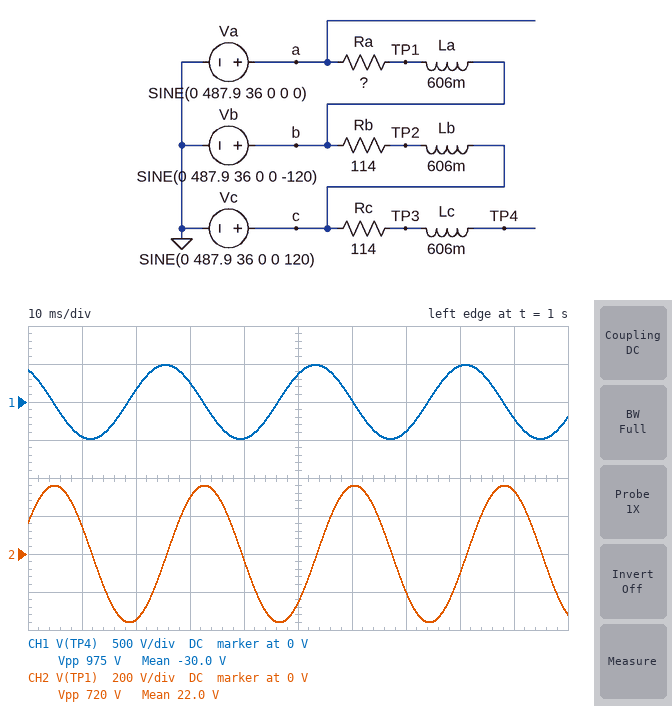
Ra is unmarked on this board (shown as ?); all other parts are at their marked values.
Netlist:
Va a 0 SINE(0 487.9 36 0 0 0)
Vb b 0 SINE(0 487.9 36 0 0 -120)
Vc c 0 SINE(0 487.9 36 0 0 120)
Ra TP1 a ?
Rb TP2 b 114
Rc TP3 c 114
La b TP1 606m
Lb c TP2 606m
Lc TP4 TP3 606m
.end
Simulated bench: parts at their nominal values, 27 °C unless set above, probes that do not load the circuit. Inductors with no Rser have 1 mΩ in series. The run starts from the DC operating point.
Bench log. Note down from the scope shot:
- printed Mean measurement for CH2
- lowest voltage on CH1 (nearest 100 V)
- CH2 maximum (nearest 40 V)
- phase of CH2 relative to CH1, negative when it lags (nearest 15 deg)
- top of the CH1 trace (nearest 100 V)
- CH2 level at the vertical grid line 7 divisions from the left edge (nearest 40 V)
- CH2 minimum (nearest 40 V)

22.0 V
-500 V
360 V
-90 deg
500 V
-200 V
-360 V
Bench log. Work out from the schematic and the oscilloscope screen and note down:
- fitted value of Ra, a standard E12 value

39 Ω
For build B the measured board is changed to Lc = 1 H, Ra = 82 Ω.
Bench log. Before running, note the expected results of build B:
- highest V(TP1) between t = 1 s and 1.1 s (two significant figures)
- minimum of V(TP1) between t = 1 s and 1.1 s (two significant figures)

240 V
-240 V
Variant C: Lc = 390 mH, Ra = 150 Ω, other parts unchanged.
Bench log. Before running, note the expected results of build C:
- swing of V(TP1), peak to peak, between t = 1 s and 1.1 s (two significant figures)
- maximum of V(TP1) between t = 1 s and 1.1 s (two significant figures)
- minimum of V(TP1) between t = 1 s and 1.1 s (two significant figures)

360 V
180 V
-180 V
